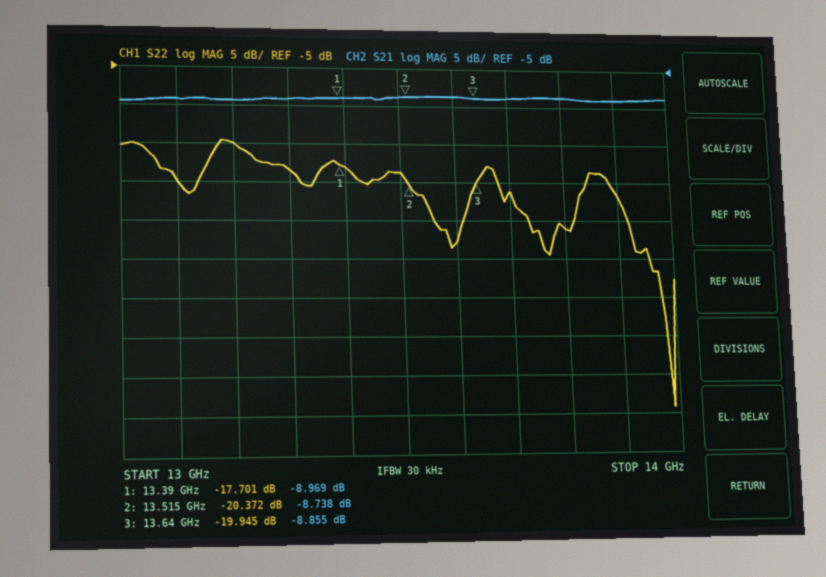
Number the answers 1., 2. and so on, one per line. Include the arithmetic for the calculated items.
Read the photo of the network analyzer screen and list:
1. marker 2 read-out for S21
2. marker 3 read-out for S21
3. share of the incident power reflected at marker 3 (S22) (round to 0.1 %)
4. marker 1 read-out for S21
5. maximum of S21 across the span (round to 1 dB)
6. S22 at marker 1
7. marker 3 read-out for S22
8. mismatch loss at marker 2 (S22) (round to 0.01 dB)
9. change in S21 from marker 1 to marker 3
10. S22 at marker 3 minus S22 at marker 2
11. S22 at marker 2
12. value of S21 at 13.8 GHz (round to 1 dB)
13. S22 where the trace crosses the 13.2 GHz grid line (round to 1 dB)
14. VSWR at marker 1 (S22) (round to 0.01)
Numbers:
1. -8.738 dB
2. -8.855 dB
3. 10^(-19.945/10) ≈ 1.0 %
4. -8.969 dB
5. -9 dB
6. -17.701 dB
7. -19.945 dB
8. −10 log10(1 − 10^(-20.372/10)) ≈ 0.04 dB
9. -8.855 − (-8.969) = 0.114 dB
10. -19.945 − (-20.372) = 0.427 dB
11. -20.372 dB
12. -9 dB
13. -15 dB
14. (1 + 0.1303)/(1 − 0.1303) ≈ 1.30
